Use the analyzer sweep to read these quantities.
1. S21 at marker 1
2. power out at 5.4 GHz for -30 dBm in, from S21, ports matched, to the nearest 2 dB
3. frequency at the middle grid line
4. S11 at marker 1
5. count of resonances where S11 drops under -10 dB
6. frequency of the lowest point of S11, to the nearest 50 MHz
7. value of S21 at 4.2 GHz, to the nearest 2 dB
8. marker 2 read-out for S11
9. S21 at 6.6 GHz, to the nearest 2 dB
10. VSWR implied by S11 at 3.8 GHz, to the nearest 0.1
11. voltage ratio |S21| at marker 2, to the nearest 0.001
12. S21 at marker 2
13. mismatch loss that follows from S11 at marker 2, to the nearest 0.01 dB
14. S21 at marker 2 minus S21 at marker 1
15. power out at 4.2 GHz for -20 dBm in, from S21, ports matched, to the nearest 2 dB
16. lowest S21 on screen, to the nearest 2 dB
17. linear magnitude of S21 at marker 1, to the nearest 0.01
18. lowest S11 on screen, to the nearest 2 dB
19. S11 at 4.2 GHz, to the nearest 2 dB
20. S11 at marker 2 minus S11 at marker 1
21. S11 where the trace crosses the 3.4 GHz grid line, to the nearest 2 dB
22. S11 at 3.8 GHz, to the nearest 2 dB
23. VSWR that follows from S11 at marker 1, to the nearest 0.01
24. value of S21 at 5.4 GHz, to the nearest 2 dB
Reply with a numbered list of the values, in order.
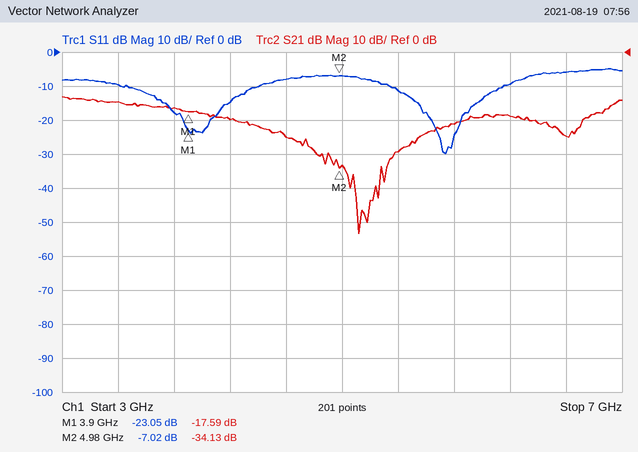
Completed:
1. -17.59 dB
2. -60 dBm
3. 5 GHz
4. -23.05 dB
5. 2
6. 5.75 GHz
7. -20 dB
8. -7.02 dB
9. -24 dB
10. 1.3
11. 0.020
12. -34.13 dB
13. 0.96 dB
14. -16.54 dB
15. -40 dBm
16. -54 dB
17. 0.13
18. -30 dB
19. -14 dB
20. 16.03 dB
21. -10 dB
22. -18 dB
23. 1.15
24. -30 dB
